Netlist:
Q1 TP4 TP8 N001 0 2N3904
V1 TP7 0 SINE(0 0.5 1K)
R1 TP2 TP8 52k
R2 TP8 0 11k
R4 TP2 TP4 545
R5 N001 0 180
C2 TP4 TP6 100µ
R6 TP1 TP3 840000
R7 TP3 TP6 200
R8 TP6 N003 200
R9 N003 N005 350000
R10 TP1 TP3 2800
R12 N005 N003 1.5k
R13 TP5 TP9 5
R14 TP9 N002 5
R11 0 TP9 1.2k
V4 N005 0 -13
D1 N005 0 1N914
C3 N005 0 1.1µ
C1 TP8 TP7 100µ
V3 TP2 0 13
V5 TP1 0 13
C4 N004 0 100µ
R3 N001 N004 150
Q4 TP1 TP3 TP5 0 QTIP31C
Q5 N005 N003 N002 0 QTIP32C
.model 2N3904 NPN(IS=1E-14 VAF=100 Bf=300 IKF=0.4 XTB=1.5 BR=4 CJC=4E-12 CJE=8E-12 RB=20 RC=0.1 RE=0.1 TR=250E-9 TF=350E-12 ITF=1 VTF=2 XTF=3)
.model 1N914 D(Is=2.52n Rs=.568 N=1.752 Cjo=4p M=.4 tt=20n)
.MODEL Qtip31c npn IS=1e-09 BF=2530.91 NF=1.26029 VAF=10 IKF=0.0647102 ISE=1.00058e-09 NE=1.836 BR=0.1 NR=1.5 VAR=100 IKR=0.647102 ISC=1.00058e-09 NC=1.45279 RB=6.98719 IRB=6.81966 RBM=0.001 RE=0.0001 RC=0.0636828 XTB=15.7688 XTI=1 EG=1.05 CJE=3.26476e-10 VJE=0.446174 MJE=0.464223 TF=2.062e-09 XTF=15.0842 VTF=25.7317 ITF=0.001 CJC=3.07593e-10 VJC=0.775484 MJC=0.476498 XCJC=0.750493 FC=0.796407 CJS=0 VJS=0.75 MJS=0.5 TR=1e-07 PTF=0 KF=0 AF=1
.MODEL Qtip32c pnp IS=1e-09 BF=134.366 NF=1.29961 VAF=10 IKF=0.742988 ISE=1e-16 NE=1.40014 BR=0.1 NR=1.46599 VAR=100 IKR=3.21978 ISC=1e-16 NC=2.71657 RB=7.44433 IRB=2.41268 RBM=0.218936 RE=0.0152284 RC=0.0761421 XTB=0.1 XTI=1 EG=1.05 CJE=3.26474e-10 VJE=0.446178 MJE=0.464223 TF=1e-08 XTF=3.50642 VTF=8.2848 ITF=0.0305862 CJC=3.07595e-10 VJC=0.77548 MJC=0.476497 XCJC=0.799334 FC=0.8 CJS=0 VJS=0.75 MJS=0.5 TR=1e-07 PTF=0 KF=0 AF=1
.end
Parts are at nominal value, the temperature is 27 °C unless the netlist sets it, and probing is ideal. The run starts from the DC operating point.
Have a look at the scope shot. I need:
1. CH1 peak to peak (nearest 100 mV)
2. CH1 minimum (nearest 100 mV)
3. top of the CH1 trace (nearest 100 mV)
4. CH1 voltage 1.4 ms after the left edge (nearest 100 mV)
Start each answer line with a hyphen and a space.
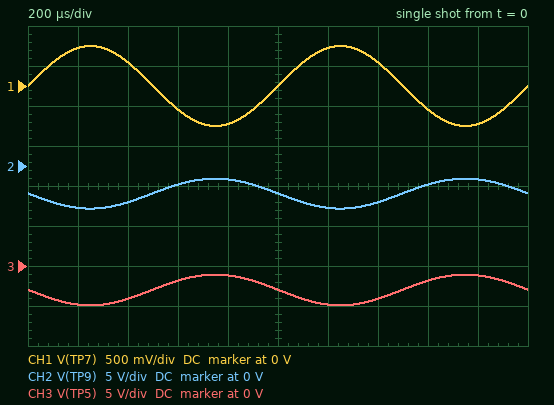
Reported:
- 1.0 V
- -500 mV
- 500 mV
- 300 mV
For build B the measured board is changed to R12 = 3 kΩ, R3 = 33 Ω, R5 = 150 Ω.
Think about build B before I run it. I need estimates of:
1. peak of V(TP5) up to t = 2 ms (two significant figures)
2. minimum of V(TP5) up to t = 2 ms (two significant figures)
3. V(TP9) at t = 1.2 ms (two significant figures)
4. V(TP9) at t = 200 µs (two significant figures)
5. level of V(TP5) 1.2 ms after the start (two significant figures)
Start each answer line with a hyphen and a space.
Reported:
- 3.9 V
- -5.3 V
- -5.4 V
- -5.5 V
- -5.1 V
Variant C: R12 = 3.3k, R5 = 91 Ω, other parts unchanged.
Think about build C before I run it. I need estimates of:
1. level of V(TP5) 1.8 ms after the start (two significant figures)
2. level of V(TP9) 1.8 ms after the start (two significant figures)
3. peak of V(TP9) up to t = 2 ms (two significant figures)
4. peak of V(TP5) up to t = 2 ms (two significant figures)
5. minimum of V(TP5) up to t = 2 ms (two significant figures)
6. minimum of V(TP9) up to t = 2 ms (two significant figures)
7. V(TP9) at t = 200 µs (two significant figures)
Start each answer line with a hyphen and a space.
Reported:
- 4.2 V
- 4.0 V
- 4.1 V
- 4.3 V
- -2.0 V
- -2.2 V
- -2.1 V
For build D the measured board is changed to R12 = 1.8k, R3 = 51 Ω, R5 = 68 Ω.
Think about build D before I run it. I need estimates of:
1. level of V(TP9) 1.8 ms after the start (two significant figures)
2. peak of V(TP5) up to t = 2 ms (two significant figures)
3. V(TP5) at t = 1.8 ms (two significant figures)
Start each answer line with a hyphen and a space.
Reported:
- 2.4 V
- 3.0 V
- 2.9 V
